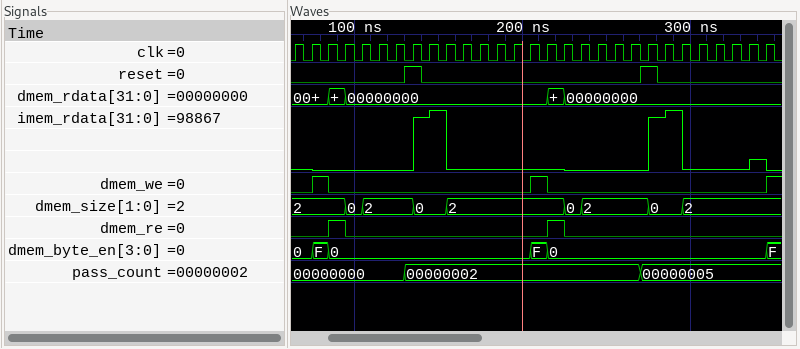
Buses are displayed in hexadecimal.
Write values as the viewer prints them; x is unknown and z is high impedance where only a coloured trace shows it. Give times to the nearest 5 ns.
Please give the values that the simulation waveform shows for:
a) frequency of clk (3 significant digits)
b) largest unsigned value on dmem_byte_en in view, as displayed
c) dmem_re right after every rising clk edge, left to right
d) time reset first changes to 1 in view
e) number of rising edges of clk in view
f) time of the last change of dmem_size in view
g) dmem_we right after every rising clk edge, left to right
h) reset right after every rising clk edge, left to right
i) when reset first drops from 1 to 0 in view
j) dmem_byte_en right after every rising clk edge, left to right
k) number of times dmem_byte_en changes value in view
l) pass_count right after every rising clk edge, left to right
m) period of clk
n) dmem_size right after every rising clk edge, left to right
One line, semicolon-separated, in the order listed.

100 MHz; F; 0 0 1 0 0 0 0 0 0 0 0 0 0 0 0 1 0 0 0 0 0 0 0 0 0 0 0 0 0; 130 ns; 29; 295 ns; 0 1 0 0 0 0 0 0 0 0 0 0 0 0 1 0 0 0 0 0 0 0 0 0 0 0 0 0 1; 0 0 0 0 0 0 0 1 0 0 0 0 0 0 0 0 0 0 0 0 0 1 0 0 0 0 0 0 0; 140 ns; 0, F, 0, 0, 0, 0, 0, 0, 0, 0, 0, 0, 0, 0, F, 0, 0, 0, 0, 0, 0, 0, 0, 0, 0, 0, 0, 0, F; 5; 00000000, 00000000, 00000000, 00000000, 00000000, 00000000, 00000000, 00000002, 00000002, 00000002, 00000002, 00000002, 00000002, 00000002, 00000002, 00000002, 00000002, 00000002, 00000002, 00000002, 00000002, 00000005, 00000005, 00000005, 00000005, 00000005, 00000005, 00000005, 00000005; 10 ns; 2, 2, 2, 0, 2, 2, 2, 0, 0, 2, 2, 2, 2, 2, 2, 2, 0, 2, 2, 2, 2, 0, 0, 2, 2, 2, 2, 2, 2
